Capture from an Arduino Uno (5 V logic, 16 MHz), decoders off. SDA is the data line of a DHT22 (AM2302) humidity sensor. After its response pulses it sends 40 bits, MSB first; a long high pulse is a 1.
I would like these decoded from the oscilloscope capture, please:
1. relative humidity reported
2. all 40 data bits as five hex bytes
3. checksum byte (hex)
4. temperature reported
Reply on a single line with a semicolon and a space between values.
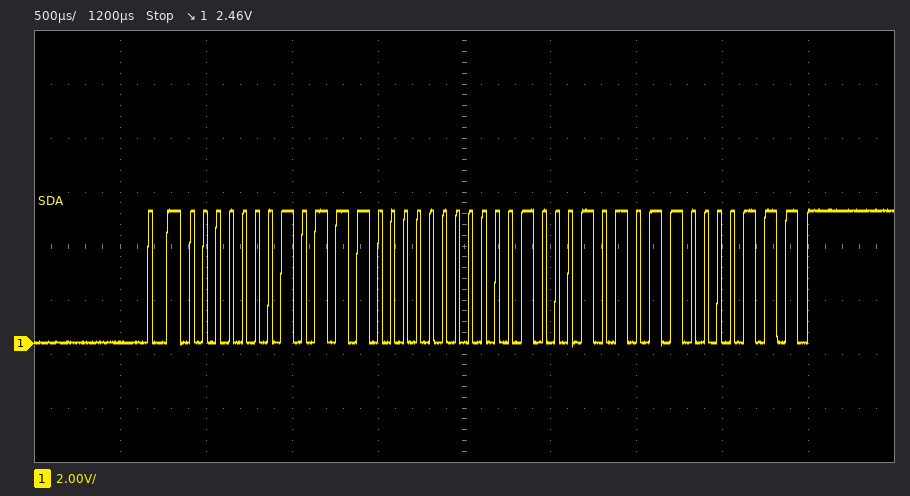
36.8 %; 01 70 01 15 87; 0x87; 27.7 °C
